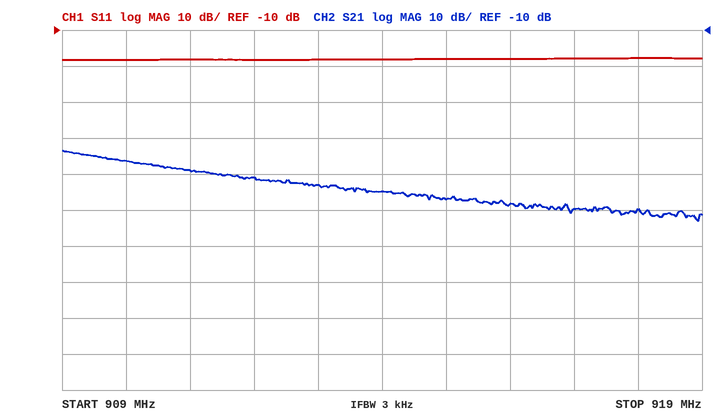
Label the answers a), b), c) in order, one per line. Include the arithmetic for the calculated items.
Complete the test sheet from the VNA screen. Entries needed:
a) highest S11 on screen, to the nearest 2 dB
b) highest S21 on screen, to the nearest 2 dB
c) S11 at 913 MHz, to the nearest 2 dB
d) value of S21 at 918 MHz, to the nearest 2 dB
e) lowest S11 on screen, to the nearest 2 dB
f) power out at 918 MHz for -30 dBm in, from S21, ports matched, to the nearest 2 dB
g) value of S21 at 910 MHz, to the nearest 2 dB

a) -18 dB
b) -44 dB
c) -18 dB
d) -60 dB
e) -18 dB
f) -30 dBm + (-60 dB) = -90 dBm
g) -46 dB
